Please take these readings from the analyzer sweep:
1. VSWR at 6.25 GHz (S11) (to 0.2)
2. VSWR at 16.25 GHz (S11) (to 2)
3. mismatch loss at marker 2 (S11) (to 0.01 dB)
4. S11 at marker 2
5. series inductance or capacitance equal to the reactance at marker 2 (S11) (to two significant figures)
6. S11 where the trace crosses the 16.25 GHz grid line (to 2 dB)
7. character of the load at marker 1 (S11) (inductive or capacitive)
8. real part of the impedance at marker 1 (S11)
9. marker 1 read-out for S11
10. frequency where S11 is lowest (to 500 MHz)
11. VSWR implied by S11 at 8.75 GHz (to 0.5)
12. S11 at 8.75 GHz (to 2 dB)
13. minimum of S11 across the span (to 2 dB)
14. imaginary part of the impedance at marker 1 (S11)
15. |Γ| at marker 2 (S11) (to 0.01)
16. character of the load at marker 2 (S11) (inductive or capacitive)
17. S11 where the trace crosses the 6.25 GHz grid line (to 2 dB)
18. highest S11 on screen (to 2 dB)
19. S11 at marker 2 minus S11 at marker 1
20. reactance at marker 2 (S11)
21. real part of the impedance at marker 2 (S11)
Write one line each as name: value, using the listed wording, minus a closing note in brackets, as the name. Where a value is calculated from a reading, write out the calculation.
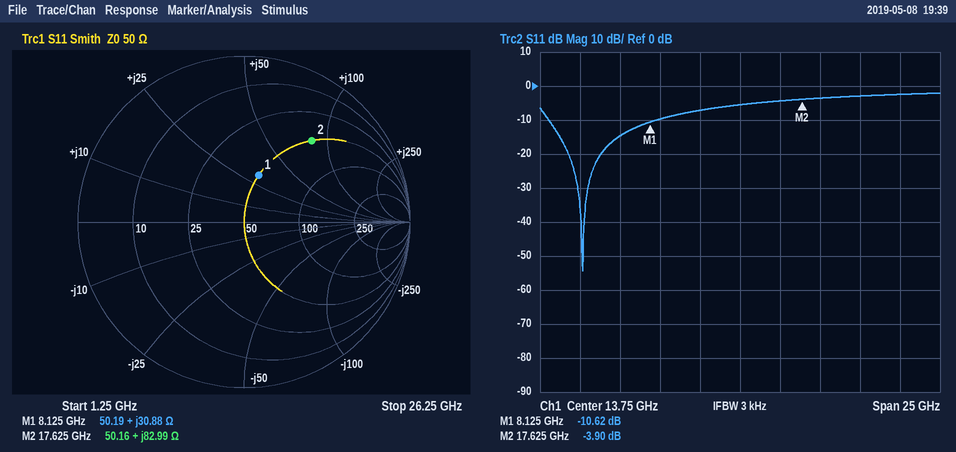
VSWR at 6.25 GHz (S11): |Γ| = 10^(-14/20) = 0.1995; VSWR = (1 + 0.1995)/(1 − 0.1995) ≈ 1.50, so 1.4 to the nearest 0.2
VSWR at 16.25 GHz (S11): |Γ| = 10^(-4/20) = 0.6310; VSWR = (1 + 0.6310)/(1 − 0.6310) ≈ 4
mismatch loss at marker 2 (S11): −10 log10(1 − 10^(-3.9/10)) ≈ 2.27 dB
S11 at marker 2: -3.90 dB
series inductance or capacitance equal to the reactance at marker 2 (S11): L = 82.99 Ω/(2π × 17.625 GHz) ≈ 749 pH, so 750 pH to two significant figures
S11 where the trace crosses the 16.25 GHz grid line: -4 dB
character of the load at marker 1 (S11): inductive
real part of the impedance at marker 1: 50.19 Ω
marker 1 read-out for S11: -10.62 dB
frequency where S11 is lowest: 4.0 GHz
VSWR implied by S11 at 8.75 GHz: |Γ| = 10^(-10/20) = 0.3162; VSWR = (1 + 0.3162)/(1 − 0.3162) ≈ 1.92, so 2.0 to the nearest 0.5
S11 at 8.75 GHz: -10 dB
minimum of S11 across the span: -54 dB
imaginary part of the impedance at marker 1: +30.88 Ω
|Γ| at marker 2 (S11): 0.64
character of the load at marker 2 (S11): inductive
S11 where the trace crosses the 6.25 GHz grid line: -14 dB
highest S11 on screen: -2 dB
S11 at marker 2 minus S11 at marker 1: -3.9 − (-10.62) = 6.72 dB
reactance at marker 2: +82.99 Ω
real part of the impedance at marker 2: 50.16 Ω
